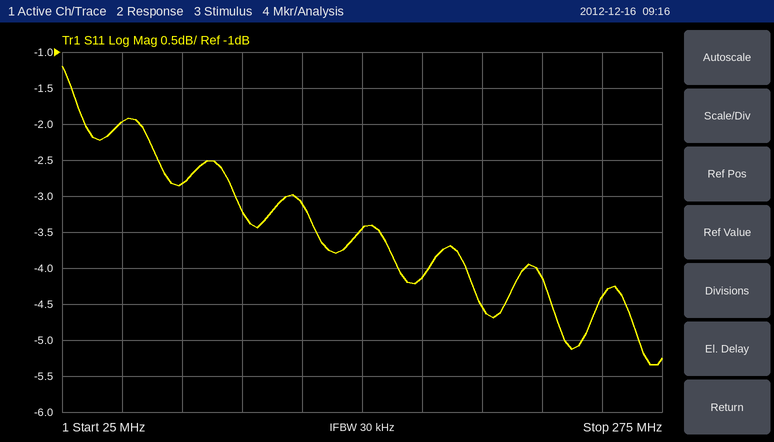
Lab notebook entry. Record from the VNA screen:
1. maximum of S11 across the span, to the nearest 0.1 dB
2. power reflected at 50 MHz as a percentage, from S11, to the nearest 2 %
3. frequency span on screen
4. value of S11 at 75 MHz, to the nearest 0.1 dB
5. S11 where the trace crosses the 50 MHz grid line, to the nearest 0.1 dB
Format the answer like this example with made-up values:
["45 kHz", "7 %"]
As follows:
["-1.2 dB", "64 %", "250 MHz", "-2.8 dB", "-2.0 dB"]
